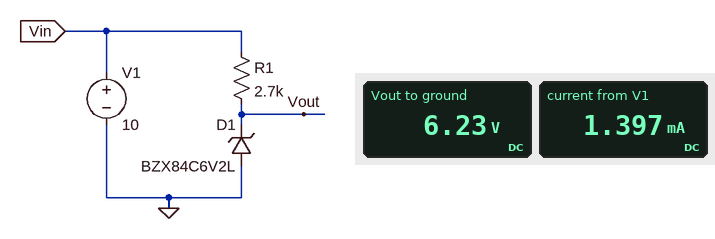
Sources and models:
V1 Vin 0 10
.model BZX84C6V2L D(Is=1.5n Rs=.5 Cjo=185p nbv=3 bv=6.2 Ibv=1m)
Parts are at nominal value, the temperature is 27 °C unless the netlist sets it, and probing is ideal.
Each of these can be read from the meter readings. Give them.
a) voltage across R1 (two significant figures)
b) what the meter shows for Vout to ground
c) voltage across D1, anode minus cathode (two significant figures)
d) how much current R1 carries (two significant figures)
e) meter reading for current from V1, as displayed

3.8 V
6.23 V
-6.2 V
1.4 mA
1.397 mA
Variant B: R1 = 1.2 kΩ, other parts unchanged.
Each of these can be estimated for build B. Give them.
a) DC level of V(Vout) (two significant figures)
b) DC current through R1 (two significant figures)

6.3 V
3.1 mA
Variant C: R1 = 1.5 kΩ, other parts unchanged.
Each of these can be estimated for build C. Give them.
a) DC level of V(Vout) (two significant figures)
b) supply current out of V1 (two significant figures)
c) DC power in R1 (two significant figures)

6.3 V
2.5 mA
9.3 mW
